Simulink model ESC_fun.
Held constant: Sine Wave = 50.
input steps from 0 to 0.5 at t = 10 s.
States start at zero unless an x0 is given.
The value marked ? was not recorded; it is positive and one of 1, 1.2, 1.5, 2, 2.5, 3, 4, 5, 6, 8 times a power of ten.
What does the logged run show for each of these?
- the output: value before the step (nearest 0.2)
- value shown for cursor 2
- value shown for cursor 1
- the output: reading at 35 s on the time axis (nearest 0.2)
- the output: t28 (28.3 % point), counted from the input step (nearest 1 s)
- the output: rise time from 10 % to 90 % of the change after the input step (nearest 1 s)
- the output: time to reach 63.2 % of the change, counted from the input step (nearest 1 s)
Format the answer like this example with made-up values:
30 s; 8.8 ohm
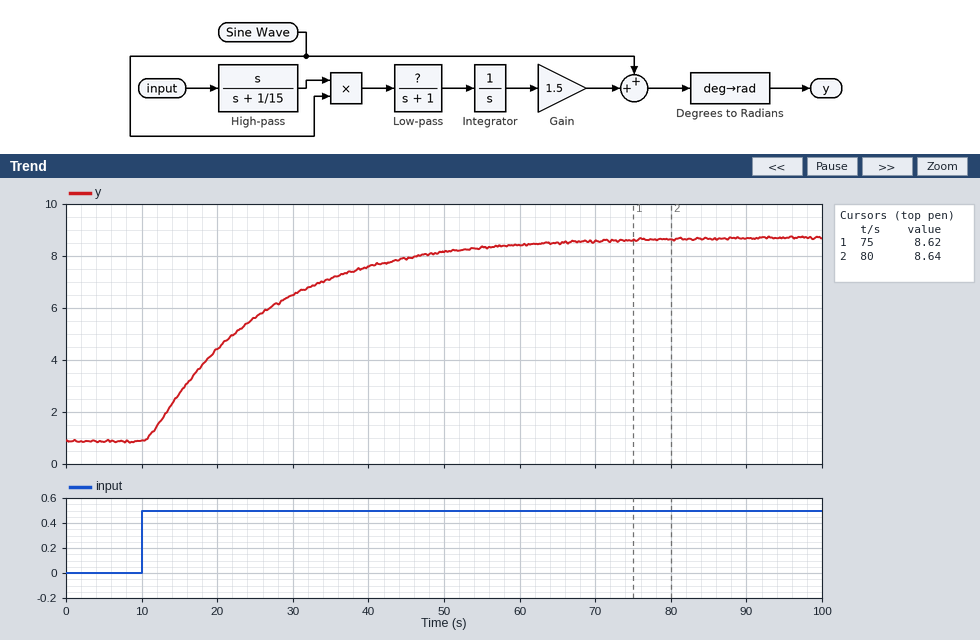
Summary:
0.8; 8.64; 8.62; 7.2; 6 s; 33 s; 16 s
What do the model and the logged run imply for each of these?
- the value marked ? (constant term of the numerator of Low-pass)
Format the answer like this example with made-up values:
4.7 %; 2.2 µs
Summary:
0.8
